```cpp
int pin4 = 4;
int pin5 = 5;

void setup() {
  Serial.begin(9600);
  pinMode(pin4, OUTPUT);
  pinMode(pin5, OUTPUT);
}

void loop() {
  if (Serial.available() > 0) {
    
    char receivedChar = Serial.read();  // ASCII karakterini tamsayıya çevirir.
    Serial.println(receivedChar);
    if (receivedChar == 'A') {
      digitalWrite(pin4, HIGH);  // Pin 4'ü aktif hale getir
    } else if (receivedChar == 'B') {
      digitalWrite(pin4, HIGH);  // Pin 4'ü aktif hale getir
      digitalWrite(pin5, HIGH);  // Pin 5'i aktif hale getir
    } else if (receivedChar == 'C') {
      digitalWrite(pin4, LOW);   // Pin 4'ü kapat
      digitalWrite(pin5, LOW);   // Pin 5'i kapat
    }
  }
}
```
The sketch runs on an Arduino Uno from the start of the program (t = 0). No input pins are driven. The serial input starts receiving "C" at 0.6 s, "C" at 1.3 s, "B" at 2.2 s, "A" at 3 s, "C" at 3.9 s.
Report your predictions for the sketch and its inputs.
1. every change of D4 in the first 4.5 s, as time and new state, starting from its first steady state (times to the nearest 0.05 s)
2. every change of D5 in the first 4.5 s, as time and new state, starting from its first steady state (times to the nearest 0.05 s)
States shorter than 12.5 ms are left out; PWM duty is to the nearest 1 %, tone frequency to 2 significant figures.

0 s low; 2.2 s high; 3.9 s low
0 s low; 2.2 s high; 3.9 s low
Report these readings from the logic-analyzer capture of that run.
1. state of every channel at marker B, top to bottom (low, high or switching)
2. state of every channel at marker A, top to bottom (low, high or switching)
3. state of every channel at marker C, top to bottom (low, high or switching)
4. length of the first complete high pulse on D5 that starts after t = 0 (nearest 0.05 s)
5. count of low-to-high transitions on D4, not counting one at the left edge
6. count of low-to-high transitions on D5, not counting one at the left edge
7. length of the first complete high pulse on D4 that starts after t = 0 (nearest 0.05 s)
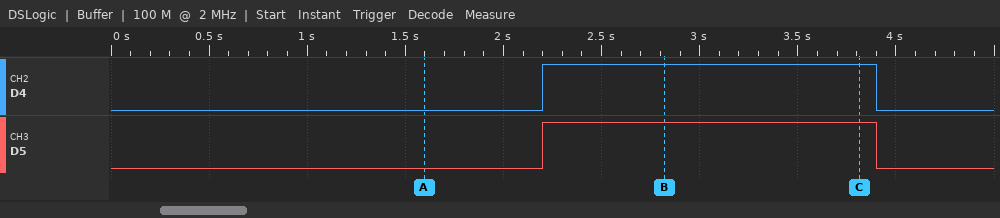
D4 high, D5 high
D4 low, D5 low
D4 high, D5 high
1.70 s
1
1
1.70 s
